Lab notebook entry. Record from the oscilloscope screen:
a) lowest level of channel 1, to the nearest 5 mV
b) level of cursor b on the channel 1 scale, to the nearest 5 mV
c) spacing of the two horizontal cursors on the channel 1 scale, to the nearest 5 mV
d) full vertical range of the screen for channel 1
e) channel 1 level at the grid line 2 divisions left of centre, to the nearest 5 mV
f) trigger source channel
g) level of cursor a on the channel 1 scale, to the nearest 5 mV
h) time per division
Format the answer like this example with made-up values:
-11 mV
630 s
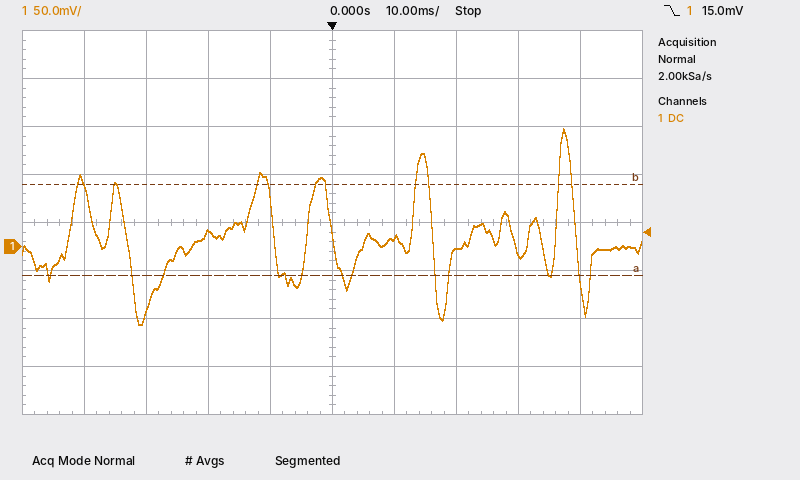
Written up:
-80 mV
65 mV
95 mV
400 mV
15 mV
channel 1
-30 mV
10 ms
